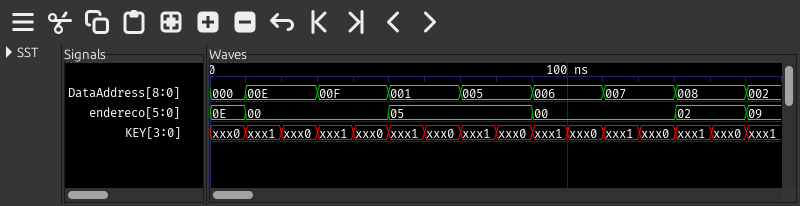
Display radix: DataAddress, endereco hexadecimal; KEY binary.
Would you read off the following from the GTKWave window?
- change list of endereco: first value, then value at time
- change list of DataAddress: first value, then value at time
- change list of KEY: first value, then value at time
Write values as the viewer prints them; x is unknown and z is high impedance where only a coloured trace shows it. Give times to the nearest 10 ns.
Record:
0E, 00 at 10 ns, 05 at 50 ns, 00 at 90 ns, 02 at 130 ns, 09 at 150 ns
000, 00E at 10 ns, 00F at 30 ns, 001 at 50 ns, 005 at 70 ns, 006 at 90 ns, 007 at 110 ns, 008 at 130 ns, 002 at 150 ns
xxx0, xxx1 at 10 ns, xxx0 at 20 ns, xxx1 at 30 ns, xxx0 at 40 ns, xxx1 at 50 ns, xxx0 at 60 ns, xxx1 at 70 ns, xxx0 at 80 ns, xxx1 at 90 ns, xxx0 at 100 ns, xxx1 at 110 ns, xxx0 at 120 ns, xxx1 at 130 ns, xxx0 at 140 ns, xxx1 at 150 ns
